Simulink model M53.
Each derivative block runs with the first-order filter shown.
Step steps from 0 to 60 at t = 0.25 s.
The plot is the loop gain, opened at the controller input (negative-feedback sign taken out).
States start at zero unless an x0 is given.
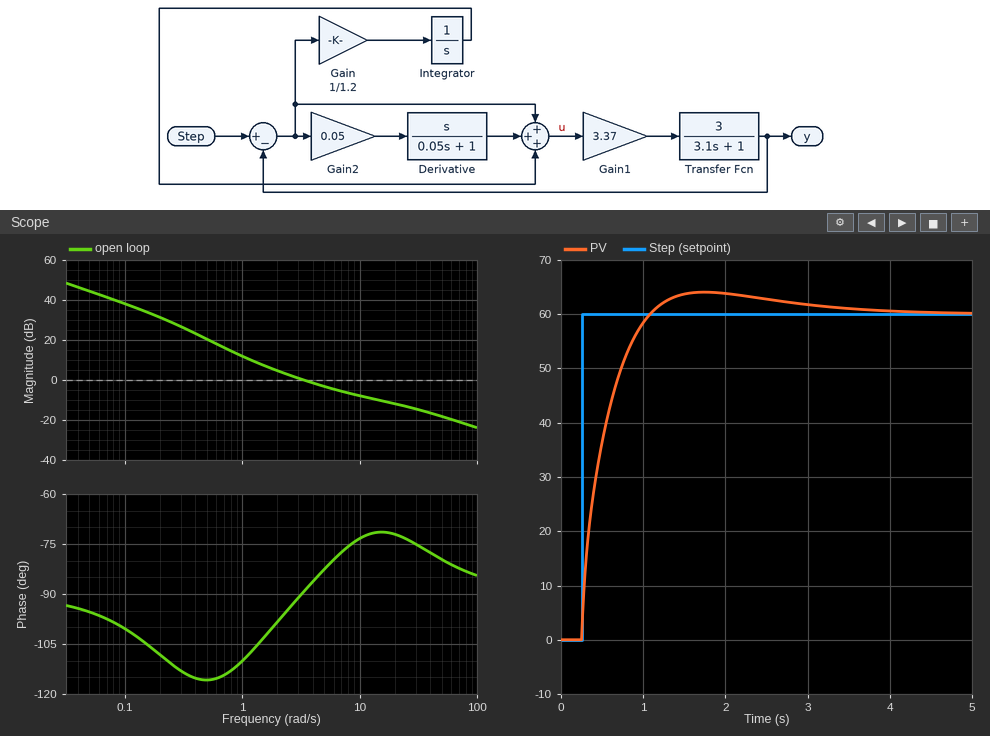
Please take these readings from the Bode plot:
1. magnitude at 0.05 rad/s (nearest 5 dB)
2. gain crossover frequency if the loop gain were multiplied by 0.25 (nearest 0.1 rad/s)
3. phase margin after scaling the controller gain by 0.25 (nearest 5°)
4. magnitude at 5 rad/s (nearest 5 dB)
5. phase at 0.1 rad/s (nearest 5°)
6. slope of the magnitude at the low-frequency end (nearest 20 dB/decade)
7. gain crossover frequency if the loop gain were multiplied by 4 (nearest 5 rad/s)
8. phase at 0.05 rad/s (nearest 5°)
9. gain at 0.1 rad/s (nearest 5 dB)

45 dB
1.0 rad/s
70°
-5 dB
-100°
-20 dB/decade
20 rad/s
-95°
40 dB
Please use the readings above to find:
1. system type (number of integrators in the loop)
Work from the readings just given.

1
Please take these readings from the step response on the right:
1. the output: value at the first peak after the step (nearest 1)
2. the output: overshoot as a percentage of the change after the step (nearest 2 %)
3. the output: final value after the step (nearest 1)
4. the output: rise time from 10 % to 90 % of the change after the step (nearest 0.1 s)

64
6 %
60
0.6 s
